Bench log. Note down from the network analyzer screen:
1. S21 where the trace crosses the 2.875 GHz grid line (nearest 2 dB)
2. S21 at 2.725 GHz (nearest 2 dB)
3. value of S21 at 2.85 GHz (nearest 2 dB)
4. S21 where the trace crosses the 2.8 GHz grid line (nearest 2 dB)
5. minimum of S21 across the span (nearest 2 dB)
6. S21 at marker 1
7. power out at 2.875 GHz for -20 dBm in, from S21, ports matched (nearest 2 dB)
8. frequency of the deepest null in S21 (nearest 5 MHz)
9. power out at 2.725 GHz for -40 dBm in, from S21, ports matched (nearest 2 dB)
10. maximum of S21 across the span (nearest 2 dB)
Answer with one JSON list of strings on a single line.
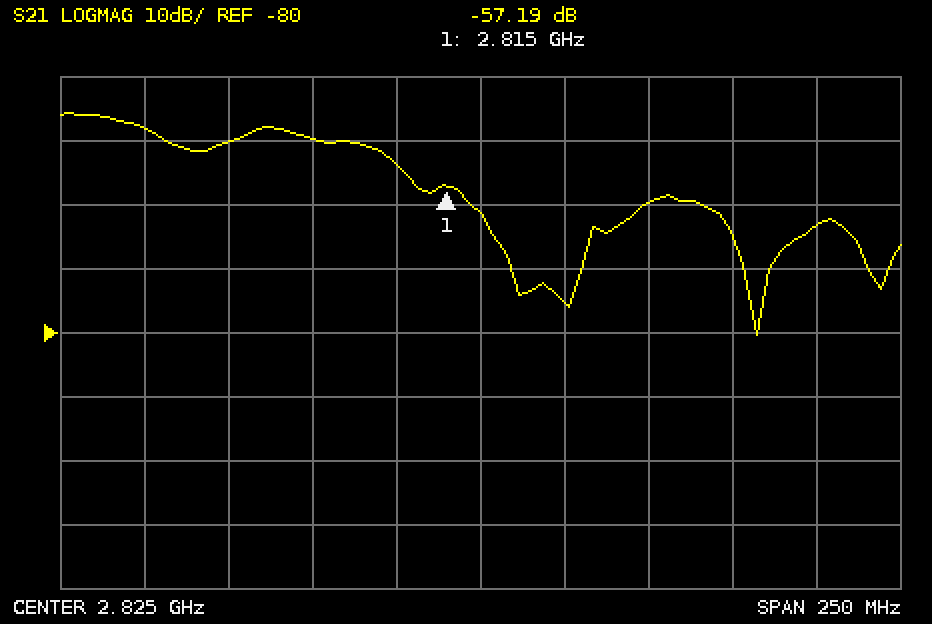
["-60 dB", "-48 dB", "-76 dB", "-54 dB", "-80 dB", "-57.19 dB", "-80 dBm", "2.905 GHz", "-88 dBm", "-46 dB"]
